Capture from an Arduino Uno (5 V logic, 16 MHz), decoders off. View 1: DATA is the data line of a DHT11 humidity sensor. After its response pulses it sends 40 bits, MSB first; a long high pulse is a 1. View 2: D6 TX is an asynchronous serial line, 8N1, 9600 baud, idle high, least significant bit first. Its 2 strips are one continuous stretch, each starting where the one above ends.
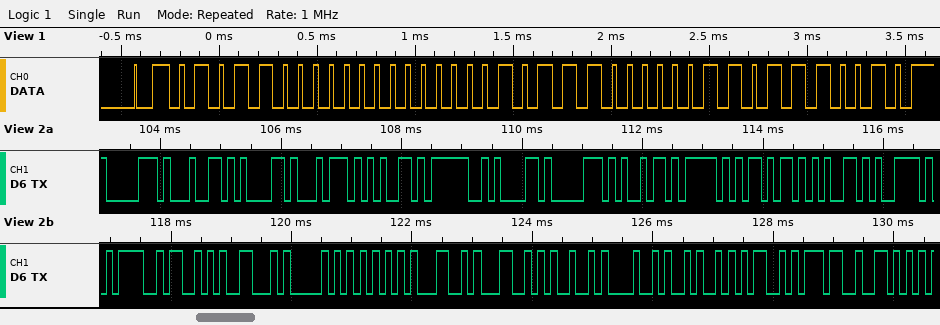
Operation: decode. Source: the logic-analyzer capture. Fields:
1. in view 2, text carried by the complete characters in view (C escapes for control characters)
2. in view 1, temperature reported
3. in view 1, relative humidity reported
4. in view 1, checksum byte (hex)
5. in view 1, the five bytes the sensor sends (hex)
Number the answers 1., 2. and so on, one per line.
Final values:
1. "pdate?api_key=SFPULLIHJM7V"
2. 23.3 °C
3. 88 %
4. 0x72
5. 58 00 17 03 72
